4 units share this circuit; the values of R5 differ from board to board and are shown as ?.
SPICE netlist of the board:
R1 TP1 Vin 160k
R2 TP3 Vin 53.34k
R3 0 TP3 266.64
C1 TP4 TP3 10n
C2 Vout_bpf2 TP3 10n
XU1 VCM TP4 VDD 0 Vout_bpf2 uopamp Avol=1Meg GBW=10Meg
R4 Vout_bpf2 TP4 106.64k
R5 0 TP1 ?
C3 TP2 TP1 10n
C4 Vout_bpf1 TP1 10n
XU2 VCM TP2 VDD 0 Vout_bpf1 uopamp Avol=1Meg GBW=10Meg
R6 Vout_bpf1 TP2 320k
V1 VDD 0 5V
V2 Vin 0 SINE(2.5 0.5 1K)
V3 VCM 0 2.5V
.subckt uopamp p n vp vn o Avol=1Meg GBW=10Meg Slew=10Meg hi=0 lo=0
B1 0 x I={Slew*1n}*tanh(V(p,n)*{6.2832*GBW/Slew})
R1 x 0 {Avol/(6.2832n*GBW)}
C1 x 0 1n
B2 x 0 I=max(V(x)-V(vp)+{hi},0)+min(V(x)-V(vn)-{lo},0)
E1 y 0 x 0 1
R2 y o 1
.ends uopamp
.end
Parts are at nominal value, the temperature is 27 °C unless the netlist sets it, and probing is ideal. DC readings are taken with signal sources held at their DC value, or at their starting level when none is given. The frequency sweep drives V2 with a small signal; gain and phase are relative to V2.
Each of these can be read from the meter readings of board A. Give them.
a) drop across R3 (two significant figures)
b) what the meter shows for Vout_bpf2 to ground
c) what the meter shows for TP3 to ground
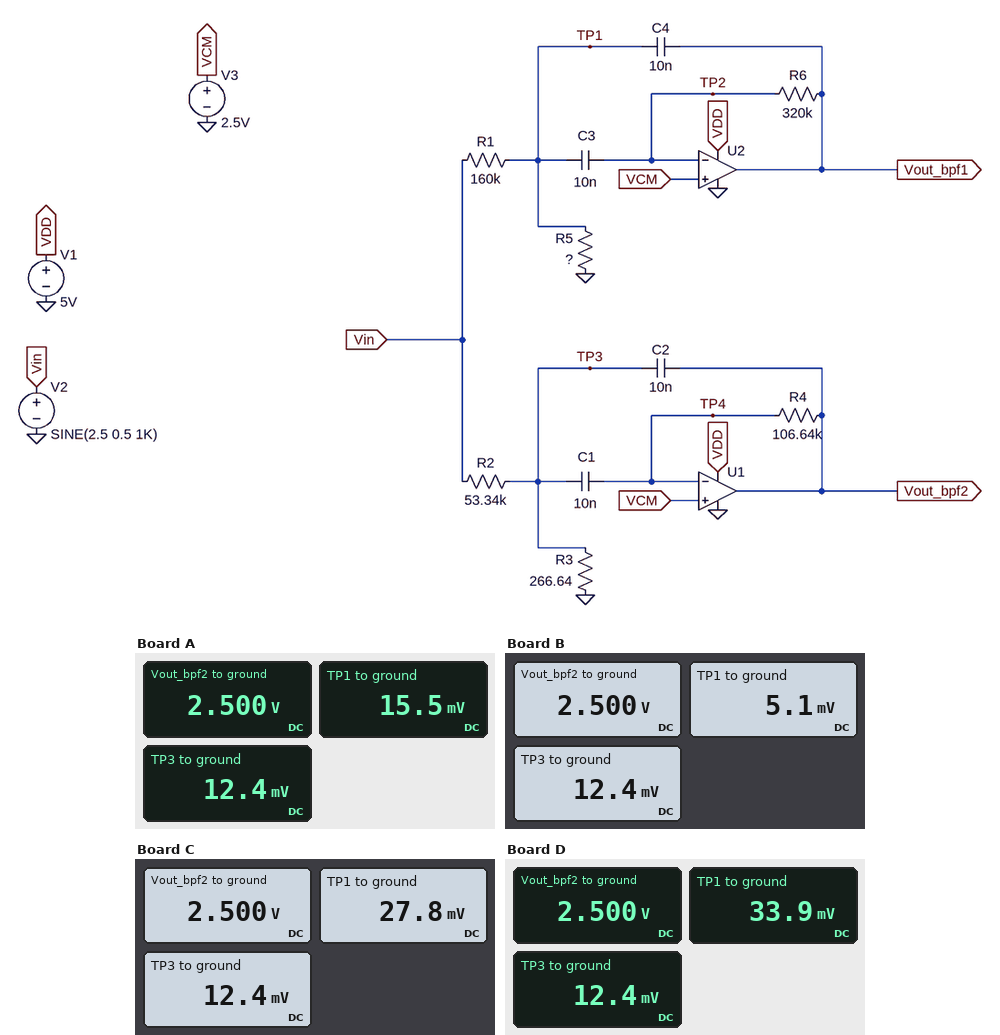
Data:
12 mV
2.500 V
12.4 mV
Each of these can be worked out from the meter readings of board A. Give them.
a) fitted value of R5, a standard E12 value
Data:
1 kΩ
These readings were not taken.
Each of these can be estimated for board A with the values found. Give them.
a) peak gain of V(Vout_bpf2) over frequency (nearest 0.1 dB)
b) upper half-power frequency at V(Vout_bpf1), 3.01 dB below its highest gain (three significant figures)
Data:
0 dB
943 Hz
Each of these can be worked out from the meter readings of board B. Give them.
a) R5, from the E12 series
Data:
330 Ω
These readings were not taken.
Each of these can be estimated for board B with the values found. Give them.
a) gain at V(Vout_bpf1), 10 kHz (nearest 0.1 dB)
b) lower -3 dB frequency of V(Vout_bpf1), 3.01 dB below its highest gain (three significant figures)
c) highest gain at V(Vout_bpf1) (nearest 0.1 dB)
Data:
-39.9 dB
1.50 kHz
0 dB
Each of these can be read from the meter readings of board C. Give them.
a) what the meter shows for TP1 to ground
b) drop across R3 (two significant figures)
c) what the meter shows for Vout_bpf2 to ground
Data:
27.8 mV
12 mV
2.500 V
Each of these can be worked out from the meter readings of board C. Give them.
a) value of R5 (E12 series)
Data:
1.8 kΩ
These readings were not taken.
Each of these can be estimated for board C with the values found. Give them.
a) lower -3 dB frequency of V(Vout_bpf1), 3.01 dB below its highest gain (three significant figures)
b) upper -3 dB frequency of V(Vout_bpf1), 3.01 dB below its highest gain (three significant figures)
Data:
619 Hz
718 Hz
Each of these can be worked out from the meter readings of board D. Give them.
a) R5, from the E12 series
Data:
2.2 kΩ
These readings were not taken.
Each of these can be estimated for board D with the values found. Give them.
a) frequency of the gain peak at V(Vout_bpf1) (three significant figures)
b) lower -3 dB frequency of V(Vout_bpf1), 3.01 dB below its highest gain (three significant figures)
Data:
604 Hz
556 Hz
